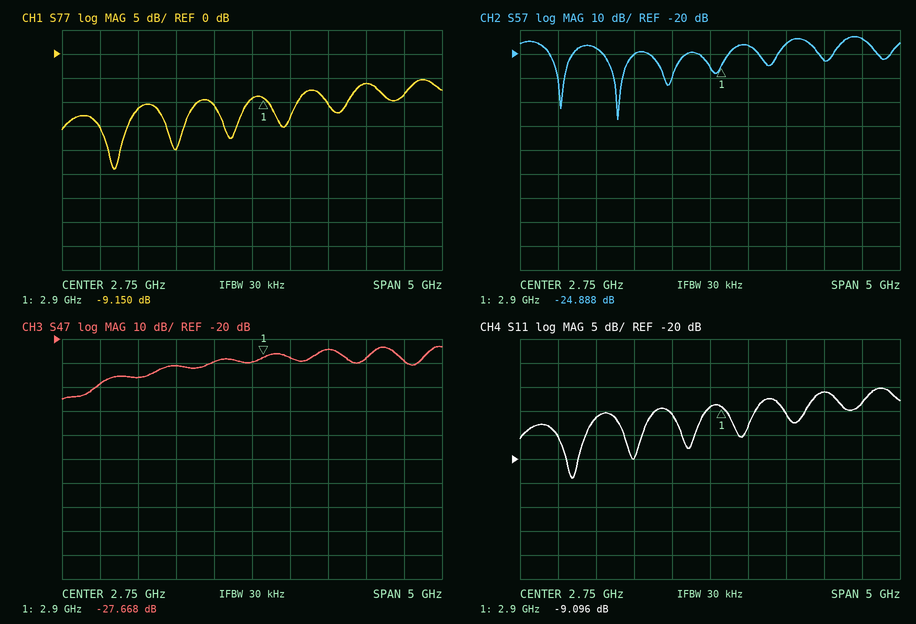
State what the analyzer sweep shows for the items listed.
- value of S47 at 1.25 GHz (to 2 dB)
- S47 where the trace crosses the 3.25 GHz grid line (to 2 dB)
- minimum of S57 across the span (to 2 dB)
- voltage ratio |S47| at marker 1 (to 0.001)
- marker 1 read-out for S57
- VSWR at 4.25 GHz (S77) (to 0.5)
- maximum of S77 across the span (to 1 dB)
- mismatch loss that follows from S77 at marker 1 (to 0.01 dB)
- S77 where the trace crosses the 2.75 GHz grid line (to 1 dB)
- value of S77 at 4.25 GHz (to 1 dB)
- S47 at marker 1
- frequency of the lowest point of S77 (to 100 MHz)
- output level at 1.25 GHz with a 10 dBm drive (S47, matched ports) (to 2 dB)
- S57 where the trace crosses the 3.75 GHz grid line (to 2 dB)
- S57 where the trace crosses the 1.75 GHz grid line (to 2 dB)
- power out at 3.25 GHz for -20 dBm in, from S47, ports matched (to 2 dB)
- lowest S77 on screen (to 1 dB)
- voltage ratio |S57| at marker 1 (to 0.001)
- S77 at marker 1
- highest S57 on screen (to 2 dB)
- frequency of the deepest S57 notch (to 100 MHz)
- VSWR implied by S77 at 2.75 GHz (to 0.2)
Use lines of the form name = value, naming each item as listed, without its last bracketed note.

value of S47 at 1.25 GHz = -36 dB
S47 where the trace crosses the 3.25 GHz grid line = -28 dB
minimum of S57 across the span = -48 dB
voltage ratio |S47| at marker 1 = 0.041
marker 1 read-out for S57 = -24.888 dB
VSWR at 4.25 GHz (S77) = 3.0
maximum of S77 across the span = -5 dB
mismatch loss that follows from S77 at marker 1 = 0.56 dB
S77 where the trace crosses the 2.75 GHz grid line = -9 dB
value of S77 at 4.25 GHz = -6 dB
S47 at marker 1 = -27.668 dB
frequency of the lowest point of S77 = 900 MHz
output level at 1.25 GHz with a 10 dBm drive (S47, matched ports) = -26 dBm
S57 where the trace crosses the 3.75 GHz grid line = -16 dB
S57 where the trace crosses the 1.75 GHz grid line = -20 dB
power out at 3.25 GHz for -20 dBm in, from S47, ports matched = -48 dBm
lowest S77 on screen = -24 dB
voltage ratio |S57| at marker 1 = 0.057
S77 at marker 1 = -9.150 dB
highest S57 on screen = -12 dB
frequency of the deepest S57 notch = 1.5 GHz
VSWR implied by S77 at 2.75 GHz = 2.0
